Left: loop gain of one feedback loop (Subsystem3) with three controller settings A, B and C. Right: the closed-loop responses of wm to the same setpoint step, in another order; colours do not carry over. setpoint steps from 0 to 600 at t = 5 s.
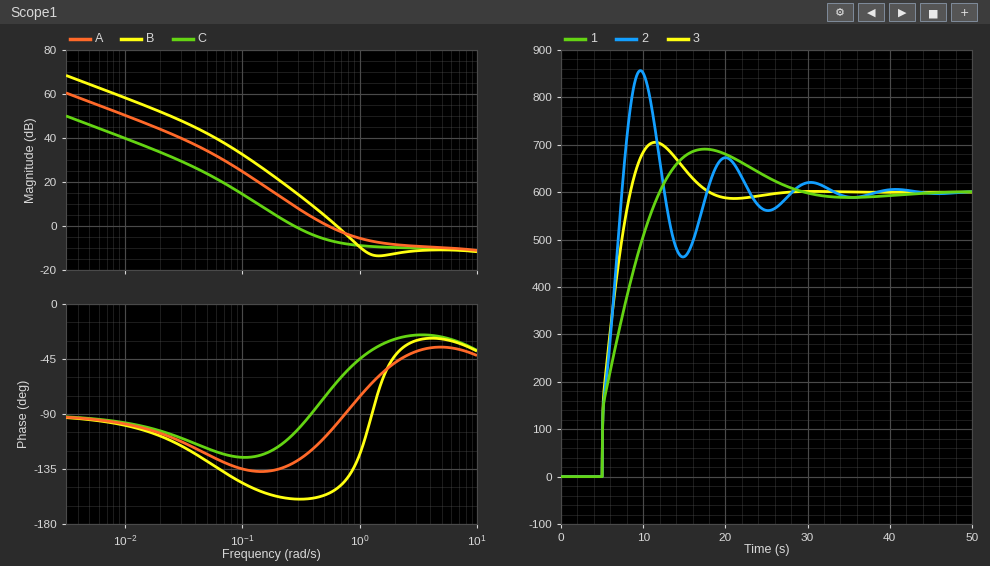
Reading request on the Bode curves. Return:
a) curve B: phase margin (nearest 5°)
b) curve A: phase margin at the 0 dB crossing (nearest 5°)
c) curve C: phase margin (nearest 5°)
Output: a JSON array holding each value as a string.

["30°", "75°", "75°"]
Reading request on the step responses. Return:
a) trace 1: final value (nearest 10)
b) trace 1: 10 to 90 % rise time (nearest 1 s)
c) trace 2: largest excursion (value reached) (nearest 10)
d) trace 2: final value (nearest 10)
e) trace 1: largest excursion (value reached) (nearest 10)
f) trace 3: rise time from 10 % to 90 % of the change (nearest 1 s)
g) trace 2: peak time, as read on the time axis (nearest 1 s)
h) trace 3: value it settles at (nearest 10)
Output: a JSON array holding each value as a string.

["600", "6 s", "860", "600", "690", "3 s", "10 s", "600"]
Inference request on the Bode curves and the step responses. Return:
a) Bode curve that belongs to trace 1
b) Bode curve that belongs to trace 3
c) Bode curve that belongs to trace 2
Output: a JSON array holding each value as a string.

["C", "A", "B"]
